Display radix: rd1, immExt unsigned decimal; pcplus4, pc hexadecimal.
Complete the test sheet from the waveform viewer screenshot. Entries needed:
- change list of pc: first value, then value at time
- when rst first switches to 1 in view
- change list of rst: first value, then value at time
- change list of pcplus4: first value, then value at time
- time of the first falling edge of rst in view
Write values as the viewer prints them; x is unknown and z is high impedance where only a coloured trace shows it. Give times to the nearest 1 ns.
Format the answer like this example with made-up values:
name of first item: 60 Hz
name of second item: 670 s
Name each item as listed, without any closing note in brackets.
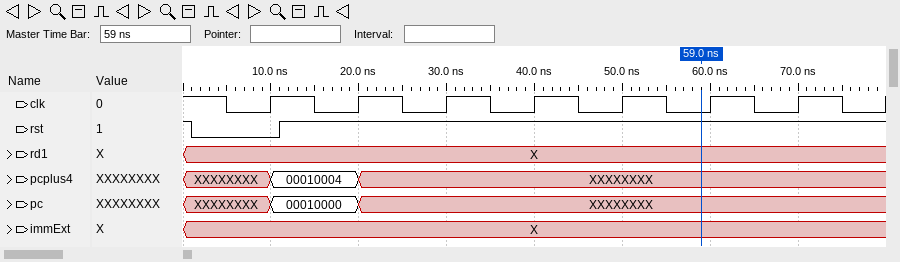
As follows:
change list of pc: first value, then value at time: XXXXXXXX, 00010000 at 10 ns, XXXXXXXX at 20 ns
when rst first switches to 1 in view: 11 ns
change list of rst: first value, then value at time: 1, 0 at 1 ns, 1 at 11 ns
change list of pcplus4: first value, then value at time: XXXXXXXX, 00010004 at 10 ns, XXXXXXXX at 20 ns
time of the first falling edge of rst in view: 1 ns
